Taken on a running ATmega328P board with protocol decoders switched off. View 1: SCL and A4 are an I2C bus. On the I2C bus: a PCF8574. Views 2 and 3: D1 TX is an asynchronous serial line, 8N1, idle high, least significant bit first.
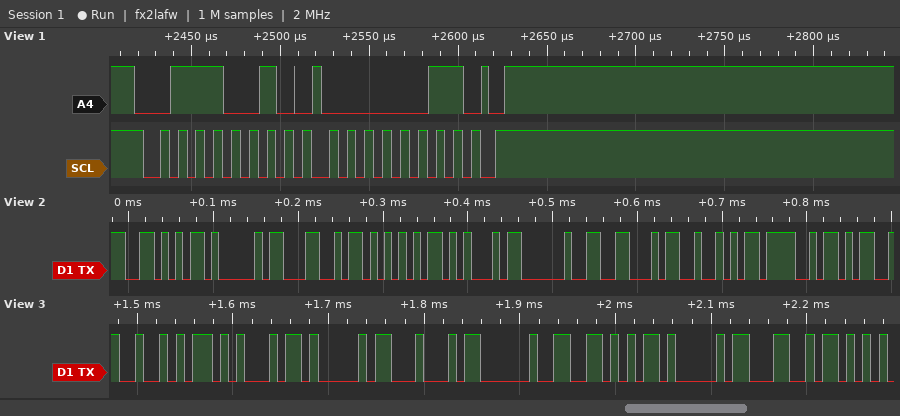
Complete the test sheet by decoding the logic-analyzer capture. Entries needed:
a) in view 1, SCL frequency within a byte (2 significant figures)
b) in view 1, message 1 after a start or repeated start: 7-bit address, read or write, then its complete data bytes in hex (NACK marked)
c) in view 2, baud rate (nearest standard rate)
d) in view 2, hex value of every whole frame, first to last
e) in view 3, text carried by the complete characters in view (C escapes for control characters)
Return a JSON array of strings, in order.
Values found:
["100 kHz", "0x39 write: 03", "115200 baud", "56 41 4C 55 45 20 46 52 4F", "\"READ VAL\""]
